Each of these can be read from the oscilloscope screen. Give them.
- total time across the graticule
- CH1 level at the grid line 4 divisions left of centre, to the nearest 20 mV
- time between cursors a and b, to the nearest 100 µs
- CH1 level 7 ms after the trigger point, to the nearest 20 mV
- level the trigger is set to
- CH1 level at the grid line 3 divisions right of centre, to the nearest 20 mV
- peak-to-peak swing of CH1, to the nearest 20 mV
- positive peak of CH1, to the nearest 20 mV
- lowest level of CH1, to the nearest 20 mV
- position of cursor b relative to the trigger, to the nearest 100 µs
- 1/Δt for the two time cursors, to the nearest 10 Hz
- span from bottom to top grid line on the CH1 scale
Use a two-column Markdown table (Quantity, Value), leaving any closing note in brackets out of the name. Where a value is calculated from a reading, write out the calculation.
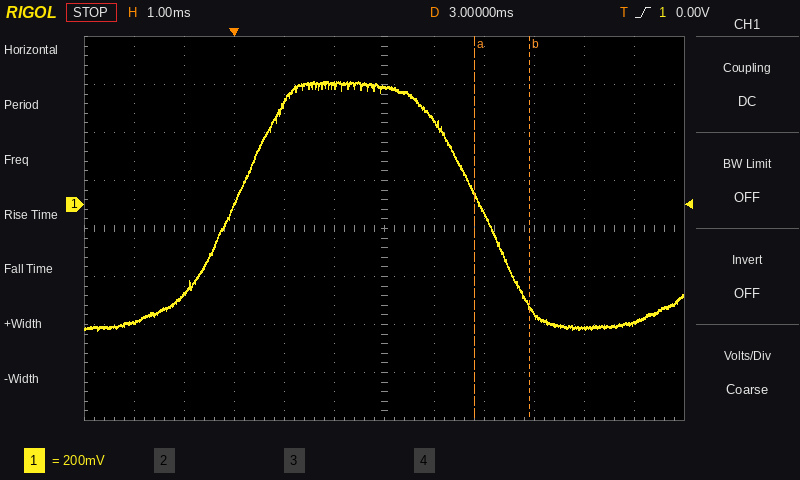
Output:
| Quantity | Value |
|---|---|
| total time across the graticule | 12 ms |
| CH1 level at the grid line 4 divisions left of centre, to the nearest 20 mV | -380 mV |
| time between cursors a and b, to the nearest 100 µs | 1.1 ms |
| CH1 level 7 ms after the trigger point, to the nearest 20 mV | -520 mV |
| level the trigger is set to | 0.00 V |
| CH1 level at the grid line 3 divisions right of centre, to the nearest 20 mV | -460 mV |
| peak-to-peak swing of CH1, to the nearest 20 mV | 520 mV − (-520 mV) = 1.04 V |
| positive peak of CH1, to the nearest 20 mV | 520 mV |
| lowest level of CH1, to the nearest 20 mV | -520 mV |
| position of cursor b relative to the trigger, to the nearest 100 µs | +5.9 ms |
| 1/Δt for the two time cursors, to the nearest 10 Hz | 1 / 1.1 ms ≈ 910 Hz |
| span from bottom to top grid line on the CH1 scale | 1.6 V |
